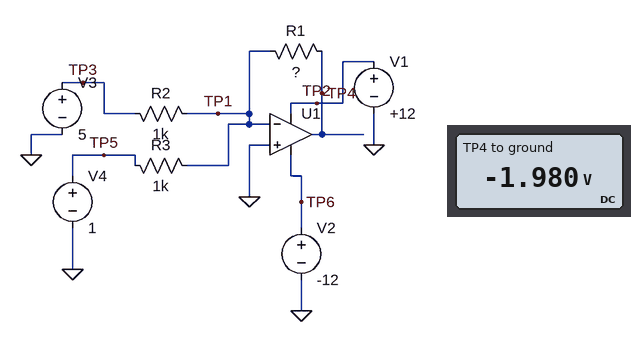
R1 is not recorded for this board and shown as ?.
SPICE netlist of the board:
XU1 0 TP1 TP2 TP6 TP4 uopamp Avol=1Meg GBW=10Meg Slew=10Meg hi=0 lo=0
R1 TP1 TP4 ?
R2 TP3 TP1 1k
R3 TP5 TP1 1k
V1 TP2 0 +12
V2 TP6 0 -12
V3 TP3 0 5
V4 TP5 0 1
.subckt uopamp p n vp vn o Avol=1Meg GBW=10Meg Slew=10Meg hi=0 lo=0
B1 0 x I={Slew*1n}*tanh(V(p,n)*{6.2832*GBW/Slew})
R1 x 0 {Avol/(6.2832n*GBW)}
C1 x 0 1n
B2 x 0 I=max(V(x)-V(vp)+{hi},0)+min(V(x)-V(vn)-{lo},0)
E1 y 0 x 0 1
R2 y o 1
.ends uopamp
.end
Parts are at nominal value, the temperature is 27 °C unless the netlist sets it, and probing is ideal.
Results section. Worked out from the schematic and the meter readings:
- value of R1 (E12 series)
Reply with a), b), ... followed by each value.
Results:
a) 330 Ω
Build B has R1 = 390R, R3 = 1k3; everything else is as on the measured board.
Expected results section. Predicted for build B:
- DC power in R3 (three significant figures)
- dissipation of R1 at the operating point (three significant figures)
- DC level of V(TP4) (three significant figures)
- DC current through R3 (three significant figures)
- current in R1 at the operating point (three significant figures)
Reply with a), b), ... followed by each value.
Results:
a) 769 µW
b) 13.0 mW
c) -2.25 V
d) 769 µA
e) 5.77 mA
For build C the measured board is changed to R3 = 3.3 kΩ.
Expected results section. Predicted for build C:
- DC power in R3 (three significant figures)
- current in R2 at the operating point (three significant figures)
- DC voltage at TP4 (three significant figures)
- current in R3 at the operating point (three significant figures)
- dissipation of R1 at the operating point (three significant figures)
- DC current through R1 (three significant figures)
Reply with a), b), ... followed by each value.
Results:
a) 303 µW
b) 5.00 mA
c) -1.75 V
d) 303 µA
e) 9.28 mW
f) 5.30 mA
